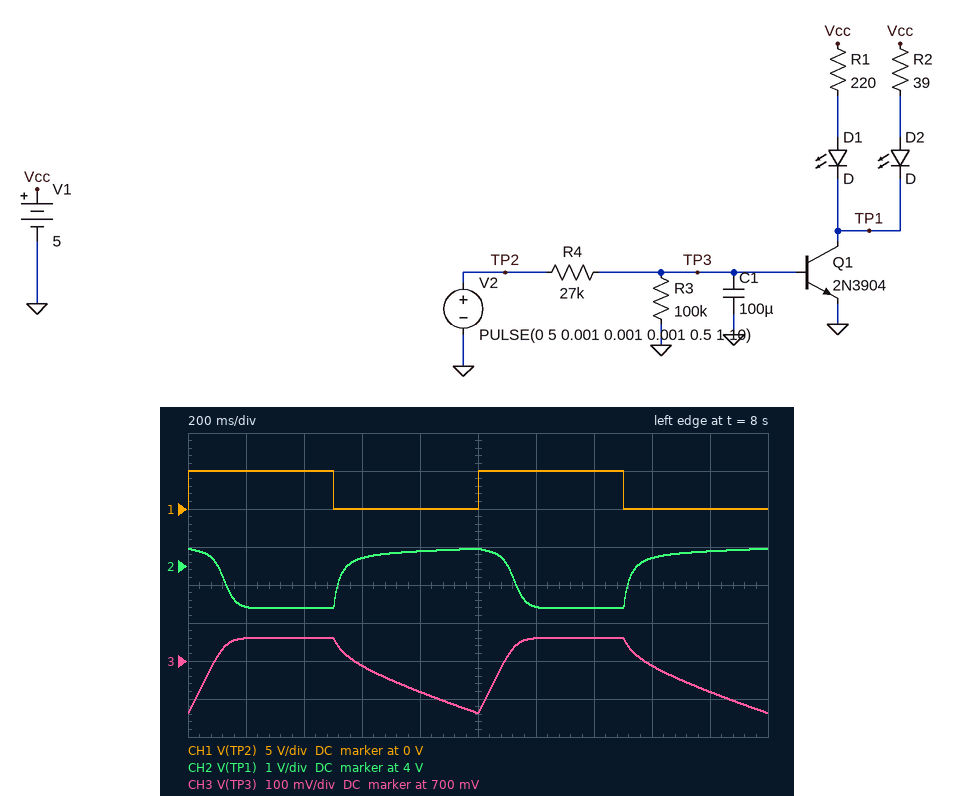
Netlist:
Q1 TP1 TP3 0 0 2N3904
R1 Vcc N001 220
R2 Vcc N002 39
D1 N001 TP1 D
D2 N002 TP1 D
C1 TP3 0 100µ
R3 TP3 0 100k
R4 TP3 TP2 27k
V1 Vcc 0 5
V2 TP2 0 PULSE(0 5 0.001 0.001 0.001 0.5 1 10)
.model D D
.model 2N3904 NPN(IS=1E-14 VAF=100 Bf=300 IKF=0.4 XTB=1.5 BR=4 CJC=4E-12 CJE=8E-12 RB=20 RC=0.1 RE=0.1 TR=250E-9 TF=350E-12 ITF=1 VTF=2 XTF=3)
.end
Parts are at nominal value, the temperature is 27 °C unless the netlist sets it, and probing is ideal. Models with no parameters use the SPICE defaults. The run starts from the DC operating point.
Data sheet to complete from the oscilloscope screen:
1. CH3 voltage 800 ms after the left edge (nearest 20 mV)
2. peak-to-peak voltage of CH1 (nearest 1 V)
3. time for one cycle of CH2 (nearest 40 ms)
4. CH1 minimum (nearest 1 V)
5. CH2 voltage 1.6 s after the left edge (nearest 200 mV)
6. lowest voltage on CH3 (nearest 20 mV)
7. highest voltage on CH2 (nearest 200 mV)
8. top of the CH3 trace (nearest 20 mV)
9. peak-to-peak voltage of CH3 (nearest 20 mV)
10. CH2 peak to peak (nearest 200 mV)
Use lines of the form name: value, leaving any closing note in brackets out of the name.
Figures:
CH3 voltage 800 ms after the left edge: 620 mV
peak-to-peak voltage of CH1: 5 V
time for one cycle of CH2: 1.00 s
CH1 minimum: 0 V
CH2 voltage 1.6 s after the left edge: 4.2 V
lowest voltage on CH3: 560 mV
highest voltage on CH2: 4.4 V
top of the CH3 trace: 760 mV
peak-to-peak voltage of CH3: 200 mV
CH2 peak to peak: 1.6 V
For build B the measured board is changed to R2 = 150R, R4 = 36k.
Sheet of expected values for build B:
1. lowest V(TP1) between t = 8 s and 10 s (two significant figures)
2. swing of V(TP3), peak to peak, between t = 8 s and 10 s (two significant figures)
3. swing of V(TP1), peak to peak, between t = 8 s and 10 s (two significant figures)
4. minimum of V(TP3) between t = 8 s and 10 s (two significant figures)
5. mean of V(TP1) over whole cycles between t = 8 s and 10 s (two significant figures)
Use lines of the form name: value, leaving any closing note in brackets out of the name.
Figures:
lowest V(TP1) between t = 8 s and 10 s: 1.5 V
swing of V(TP3), peak to peak, between t = 8 s and 10 s: 170 mV
swing of V(TP1), peak to peak, between t = 8 s and 10 s: 2.9 V
minimum of V(TP3) between t = 8 s and 10 s: 580 mV
mean of V(TP1) over whole cycles between t = 8 s and 10 s: 3.2 V
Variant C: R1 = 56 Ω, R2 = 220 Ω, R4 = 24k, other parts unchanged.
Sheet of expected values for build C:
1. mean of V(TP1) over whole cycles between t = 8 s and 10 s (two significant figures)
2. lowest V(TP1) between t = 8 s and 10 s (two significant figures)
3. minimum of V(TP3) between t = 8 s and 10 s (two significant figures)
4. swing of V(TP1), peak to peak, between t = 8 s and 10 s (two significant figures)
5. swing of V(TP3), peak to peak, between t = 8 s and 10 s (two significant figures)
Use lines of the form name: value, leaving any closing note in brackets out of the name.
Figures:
mean of V(TP1) over whole cycles between t = 8 s and 10 s: 3.5 V
lowest V(TP1) between t = 8 s and 10 s: 2.2 V
minimum of V(TP3) between t = 8 s and 10 s: 550 mV
swing of V(TP1), peak to peak, between t = 8 s and 10 s: 2.3 V
swing of V(TP3), peak to peak, between t = 8 s and 10 s: 210 mV
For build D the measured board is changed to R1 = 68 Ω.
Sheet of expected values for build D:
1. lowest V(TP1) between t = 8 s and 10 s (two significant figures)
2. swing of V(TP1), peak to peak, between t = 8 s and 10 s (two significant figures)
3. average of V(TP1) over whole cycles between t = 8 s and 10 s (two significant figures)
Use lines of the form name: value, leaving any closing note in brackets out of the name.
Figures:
lowest V(TP1) between t = 8 s and 10 s: 3.2 V
swing of V(TP1), peak to peak, between t = 8 s and 10 s: 1.2 V
average of V(TP1) over whole cycles between t = 8 s and 10 s: 3.9 V
